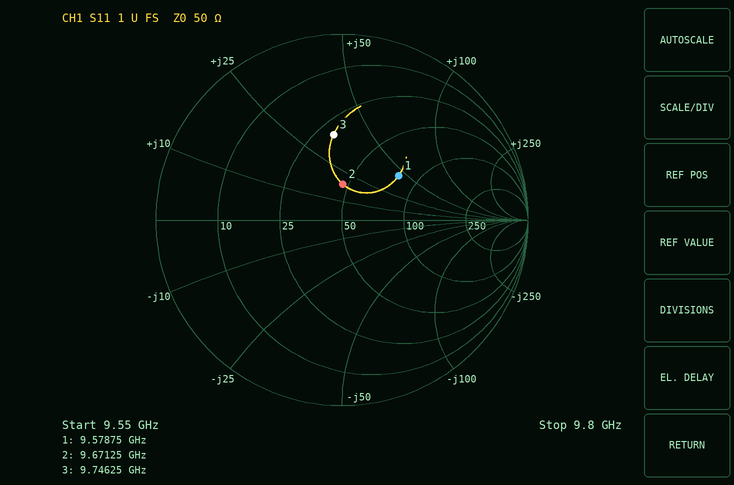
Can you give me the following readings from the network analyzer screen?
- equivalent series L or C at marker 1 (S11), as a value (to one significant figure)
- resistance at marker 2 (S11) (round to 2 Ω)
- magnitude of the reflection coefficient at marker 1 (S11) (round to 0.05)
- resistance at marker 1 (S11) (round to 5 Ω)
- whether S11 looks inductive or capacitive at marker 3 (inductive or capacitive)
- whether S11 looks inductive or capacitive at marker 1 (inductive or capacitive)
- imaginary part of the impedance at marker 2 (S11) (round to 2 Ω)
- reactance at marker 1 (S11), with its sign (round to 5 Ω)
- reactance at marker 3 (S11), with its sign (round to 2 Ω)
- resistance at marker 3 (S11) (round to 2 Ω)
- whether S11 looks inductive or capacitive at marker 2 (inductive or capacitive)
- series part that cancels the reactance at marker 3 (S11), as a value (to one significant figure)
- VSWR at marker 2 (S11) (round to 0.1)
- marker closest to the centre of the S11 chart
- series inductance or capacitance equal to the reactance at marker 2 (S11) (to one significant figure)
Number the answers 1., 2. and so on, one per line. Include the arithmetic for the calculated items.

1. L = 45 Ω/(2π × 9.57875 GHz) ≈ 748 pH, so 700 pH to one significant figure
2. 46 Ω
3. 0.40
4. 80 Ω
5. inductive
6. inductive
7. +18 Ω
8. +45 Ω
9. +36 Ω
10. 30 Ω
11. inductive
12. C = 1/(2π × 9.74625 GHz × 36 Ω) ≈ 454 fF, so 500 fF to one significant figure
13. 1.5
14. marker 2
15. L = 18 Ω/(2π × 9.67125 GHz) ≈ 296 pH, so 300 pH to one significant figure
